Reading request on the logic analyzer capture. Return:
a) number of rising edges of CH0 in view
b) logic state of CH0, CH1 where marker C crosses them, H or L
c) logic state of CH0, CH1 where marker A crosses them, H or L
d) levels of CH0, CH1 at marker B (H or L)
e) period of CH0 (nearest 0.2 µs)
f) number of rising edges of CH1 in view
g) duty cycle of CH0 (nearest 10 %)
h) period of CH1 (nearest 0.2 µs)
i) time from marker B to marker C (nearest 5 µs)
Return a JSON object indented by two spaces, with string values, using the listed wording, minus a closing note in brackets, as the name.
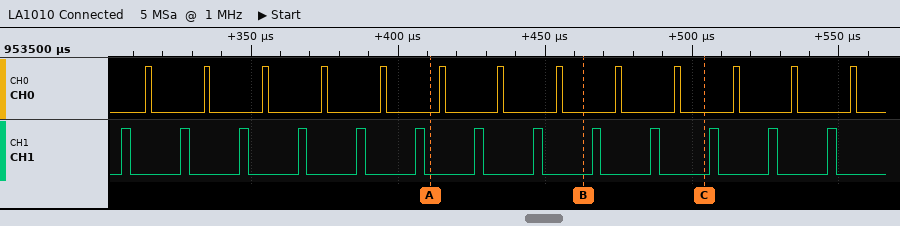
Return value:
{
  "number of rising edges of CH0 in view": "13",
  "logic state of CH0, CH1 where marker C crosses them, H or L": "CH0=L, CH1=L",
  "logic state of CH0, CH1 where marker A crosses them, H or L": "CH0=L, CH1=L",
  "levels of CH0, CH1 at marker B": "CH0=L, CH1=L",
  "period of CH0": "20 µs",
  "number of rising edges of CH1 in view": "13",
  "duty cycle of CH0": "10 %",
  "period of CH1": "20 µs",
  "time from marker B to marker C": "40 µs"
}
